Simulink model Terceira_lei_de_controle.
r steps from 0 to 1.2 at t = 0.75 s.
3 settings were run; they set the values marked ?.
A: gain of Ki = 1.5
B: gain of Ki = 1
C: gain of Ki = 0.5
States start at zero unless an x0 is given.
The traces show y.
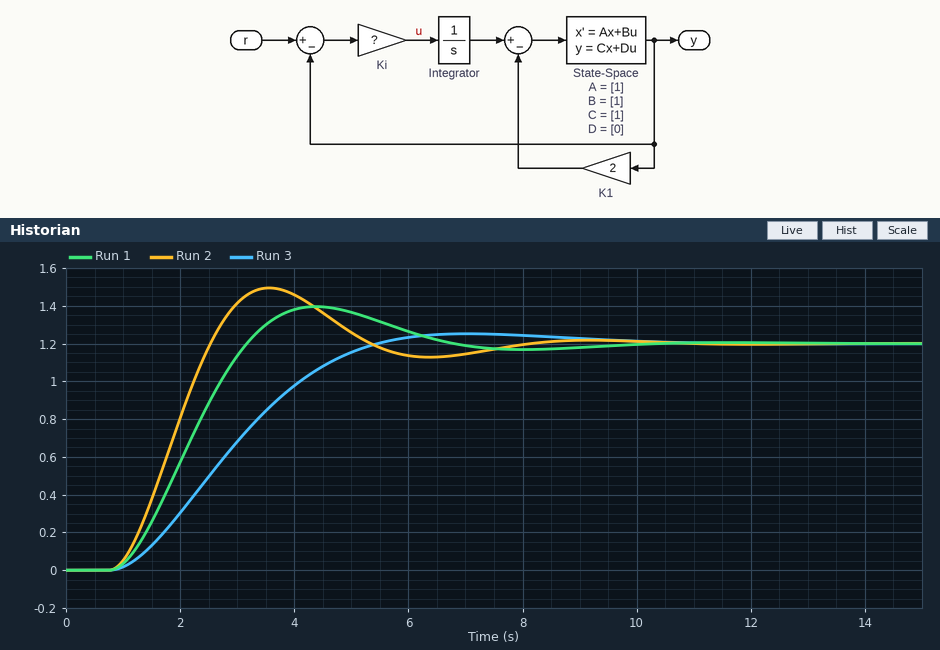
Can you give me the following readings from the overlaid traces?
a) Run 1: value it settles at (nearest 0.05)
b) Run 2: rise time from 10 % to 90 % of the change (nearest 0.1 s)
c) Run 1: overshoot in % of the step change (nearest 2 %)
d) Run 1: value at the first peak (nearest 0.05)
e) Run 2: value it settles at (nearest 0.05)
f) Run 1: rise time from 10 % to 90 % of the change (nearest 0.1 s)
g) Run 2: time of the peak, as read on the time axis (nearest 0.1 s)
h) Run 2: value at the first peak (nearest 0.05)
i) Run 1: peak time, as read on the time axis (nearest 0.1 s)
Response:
1.20
1.2 s
16 %
1.40
1.20
1.6 s
3.6 s
1.50
4.4 s
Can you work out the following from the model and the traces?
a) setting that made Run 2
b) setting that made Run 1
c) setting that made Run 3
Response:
A
B
C
